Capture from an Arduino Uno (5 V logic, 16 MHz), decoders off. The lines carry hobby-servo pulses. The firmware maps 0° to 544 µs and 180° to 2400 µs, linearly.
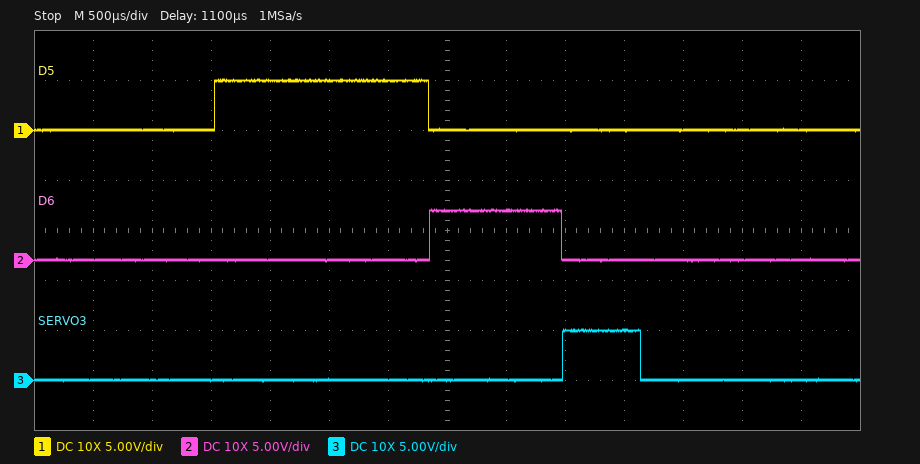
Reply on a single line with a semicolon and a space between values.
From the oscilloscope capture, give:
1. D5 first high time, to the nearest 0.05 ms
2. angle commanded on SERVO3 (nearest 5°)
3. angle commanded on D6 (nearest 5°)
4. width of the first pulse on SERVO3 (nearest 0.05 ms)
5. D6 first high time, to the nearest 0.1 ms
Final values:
1.80 ms; 10°; 55°; 0.65 ms; 1.1 ms
